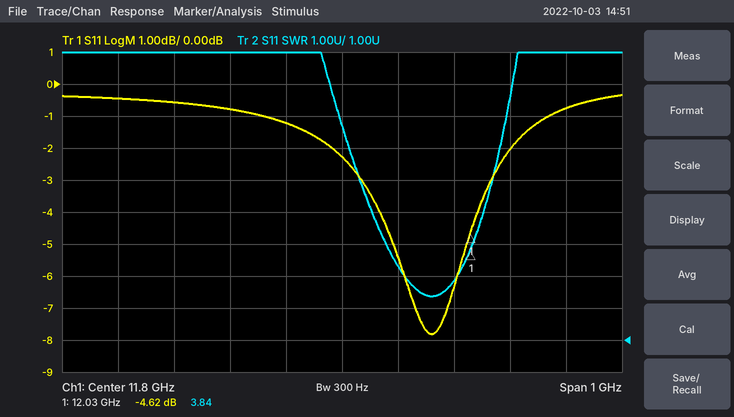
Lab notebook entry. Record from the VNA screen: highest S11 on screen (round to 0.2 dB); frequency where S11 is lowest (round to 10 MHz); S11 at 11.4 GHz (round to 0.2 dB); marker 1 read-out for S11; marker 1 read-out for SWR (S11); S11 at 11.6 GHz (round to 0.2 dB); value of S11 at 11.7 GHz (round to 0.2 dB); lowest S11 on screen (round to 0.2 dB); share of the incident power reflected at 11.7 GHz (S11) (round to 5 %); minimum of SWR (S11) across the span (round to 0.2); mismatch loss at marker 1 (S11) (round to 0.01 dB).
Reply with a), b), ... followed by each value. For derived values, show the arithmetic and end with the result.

a) -0.4 dB
b) 11.96 GHz
c) -0.4 dB
d) -4.62 dB
e) 3.84
f) -0.8 dB
g) -1.2 dB
h) -7.8 dB
i) 10^(-1.2/10) ≈ 75.9 %, so 75 % to the nearest 5 %
j) 2.4
k) −10 log10(1 − 10^(-4.62/10)) ≈ 1.84 dB
